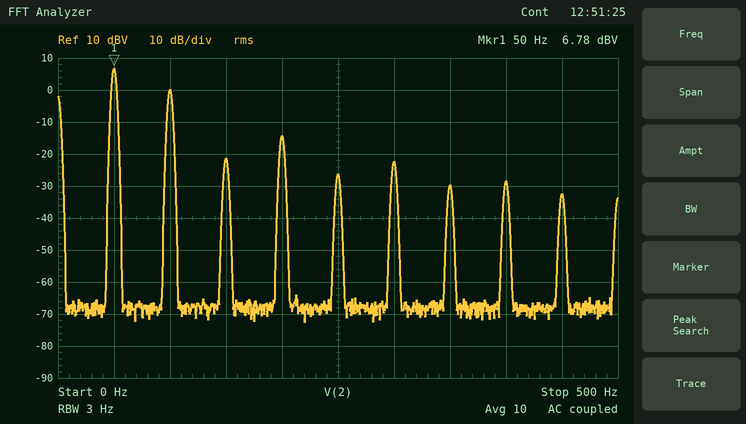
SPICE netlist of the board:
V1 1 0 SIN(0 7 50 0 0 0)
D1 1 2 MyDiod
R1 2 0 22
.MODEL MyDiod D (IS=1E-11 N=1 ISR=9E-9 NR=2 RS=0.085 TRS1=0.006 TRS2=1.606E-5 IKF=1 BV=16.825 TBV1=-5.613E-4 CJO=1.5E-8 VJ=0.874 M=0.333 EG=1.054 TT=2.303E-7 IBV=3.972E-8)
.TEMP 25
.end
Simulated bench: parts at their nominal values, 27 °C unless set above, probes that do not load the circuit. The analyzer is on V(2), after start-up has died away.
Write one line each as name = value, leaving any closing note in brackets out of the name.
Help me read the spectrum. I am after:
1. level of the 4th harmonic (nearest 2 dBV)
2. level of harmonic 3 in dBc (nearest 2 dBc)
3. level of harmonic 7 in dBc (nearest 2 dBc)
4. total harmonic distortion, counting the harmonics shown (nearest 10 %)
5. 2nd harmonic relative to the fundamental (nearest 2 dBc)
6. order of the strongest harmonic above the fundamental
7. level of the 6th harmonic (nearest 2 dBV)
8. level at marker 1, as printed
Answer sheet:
level of the 4th harmonic = -14 dBV
level of harmonic 3 in dBc = -28 dBc
level of harmonic 7 in dBc = -36 dBc
total harmonic distortion, counting the harmonics shown = 50 %
2nd harmonic relative to the fundamental = -6 dBc
order of the strongest harmonic above the fundamental = 2
level of the 6th harmonic = -22 dBV
level at marker 1, as printed = 6.78 dBV
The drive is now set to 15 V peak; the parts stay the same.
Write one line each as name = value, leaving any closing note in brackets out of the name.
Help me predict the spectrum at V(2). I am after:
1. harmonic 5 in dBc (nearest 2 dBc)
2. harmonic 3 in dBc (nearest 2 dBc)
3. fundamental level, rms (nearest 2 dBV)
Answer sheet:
harmonic 5 in dBc = -40 dBc
harmonic 3 in dBc = -34 dBc
fundamental level, rms = 14 dBV
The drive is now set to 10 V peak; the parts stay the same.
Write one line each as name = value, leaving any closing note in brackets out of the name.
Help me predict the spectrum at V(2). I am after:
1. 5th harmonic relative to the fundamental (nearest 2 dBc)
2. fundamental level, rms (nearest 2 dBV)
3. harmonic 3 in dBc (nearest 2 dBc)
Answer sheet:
5th harmonic relative to the fundamental = -36 dBc
fundamental level, rms = 10 dBV
harmonic 3 in dBc = -32 dBc
